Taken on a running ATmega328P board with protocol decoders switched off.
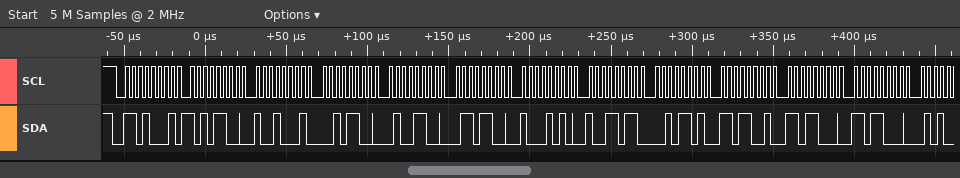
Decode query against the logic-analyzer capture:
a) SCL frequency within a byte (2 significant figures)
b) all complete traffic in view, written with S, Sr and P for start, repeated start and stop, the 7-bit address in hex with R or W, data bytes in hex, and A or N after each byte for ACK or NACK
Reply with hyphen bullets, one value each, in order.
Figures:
- 250 kHz
- S 68R A AC A 91 A 2C A 4C A 6C A 8A A 9B A 2D A D9 A D8 A D8 A
